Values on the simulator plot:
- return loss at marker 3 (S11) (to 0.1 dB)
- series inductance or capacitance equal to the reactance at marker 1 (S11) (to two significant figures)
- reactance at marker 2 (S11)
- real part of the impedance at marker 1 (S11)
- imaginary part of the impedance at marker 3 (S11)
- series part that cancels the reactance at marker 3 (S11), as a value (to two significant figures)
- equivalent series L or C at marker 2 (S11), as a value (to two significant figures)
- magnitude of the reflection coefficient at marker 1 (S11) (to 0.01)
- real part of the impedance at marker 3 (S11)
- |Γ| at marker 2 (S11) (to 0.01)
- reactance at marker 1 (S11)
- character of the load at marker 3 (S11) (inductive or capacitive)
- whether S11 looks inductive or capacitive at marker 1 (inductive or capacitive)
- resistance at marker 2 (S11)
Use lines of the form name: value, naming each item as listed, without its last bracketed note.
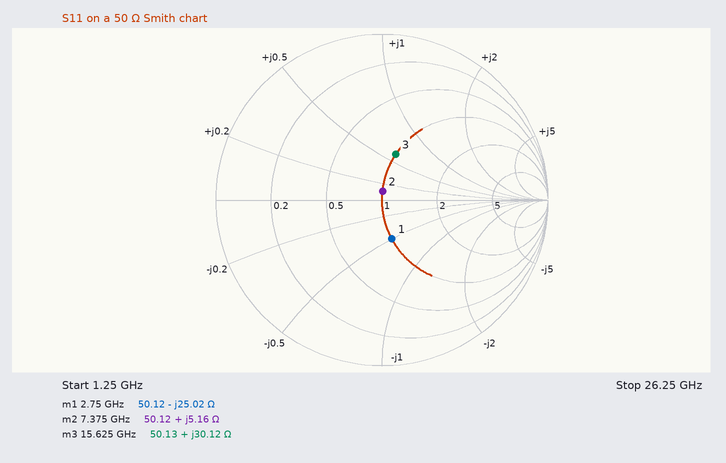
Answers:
return loss at marker 3 (S11): 10.8 dB
series inductance or capacitance equal to the reactance at marker 1 (S11): 2.3 pF
reactance at marker 2: +5.16 Ω
real part of the impedance at marker 1: 50.12 Ω
imaginary part of the impedance at marker 3: +30.12 Ω
series part that cancels the reactance at marker 3 (S11), as a value: 340 fF
equivalent series L or C at marker 2 (S11), as a value: 110 pH
magnitude of the reflection coefficient at marker 1 (S11): 0.24
real part of the impedance at marker 3: 50.13 Ω
|Γ| at marker 2 (S11): 0.05
reactance at marker 1: -25.02 Ω
character of the load at marker 3 (S11): inductive
whether S11 looks inductive or capacitive at marker 1: capacitive
resistance at marker 2: 50.12 Ω
